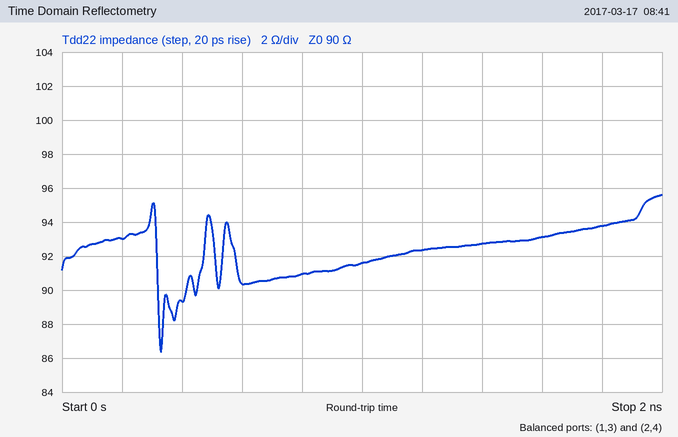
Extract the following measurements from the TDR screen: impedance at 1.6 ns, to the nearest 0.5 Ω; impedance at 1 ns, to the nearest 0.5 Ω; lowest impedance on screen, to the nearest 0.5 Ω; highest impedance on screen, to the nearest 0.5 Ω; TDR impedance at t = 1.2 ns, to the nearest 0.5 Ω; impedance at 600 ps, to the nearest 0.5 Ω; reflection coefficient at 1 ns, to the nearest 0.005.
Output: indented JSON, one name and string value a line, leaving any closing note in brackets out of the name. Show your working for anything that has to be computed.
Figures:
{
  "impedance at 1.6 ns, to the nearest 0.5 Ω": "93.0 Ω",
  "impedance at 1 ns, to the nearest 0.5 Ω": "91.5 Ω",
  "lowest impedance on screen, to the nearest 0.5 Ω": "86.5 Ω",
  "highest impedance on screen, to the nearest 0.5 Ω": "95.5 Ω",
  "TDR impedance at t = 1.2 ns, to the nearest 0.5 Ω": "92.5 Ω",
  "impedance at 600 ps, to the nearest 0.5 Ω": "90.5 Ω",
  "reflection coefficient at 1 ns, to the nearest 0.005": "(91.5 − 90)/(91.5 + 90) ≈ +0.00826, so +0.010 to the nearest 0.005"
}
